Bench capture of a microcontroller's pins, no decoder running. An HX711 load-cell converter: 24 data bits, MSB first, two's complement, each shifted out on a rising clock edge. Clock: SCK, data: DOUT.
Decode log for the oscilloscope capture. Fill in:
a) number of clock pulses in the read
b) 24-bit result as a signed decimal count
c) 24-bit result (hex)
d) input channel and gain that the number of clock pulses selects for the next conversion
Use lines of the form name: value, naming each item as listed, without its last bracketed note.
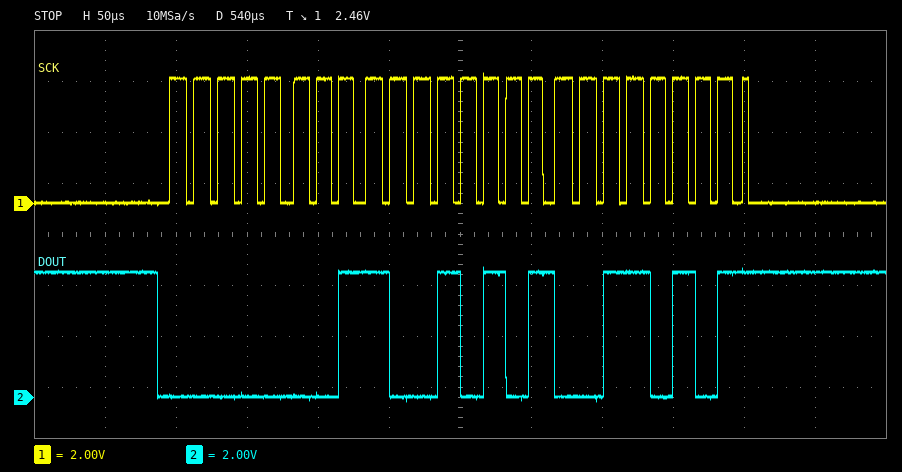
number of clock pulses in the read: 25
24-bit result as a signed decimal count: 103733
24-bit result: 0x019535
input channel and gain that the number of clock pulses selects for the next conversion: channel A, gain 128
